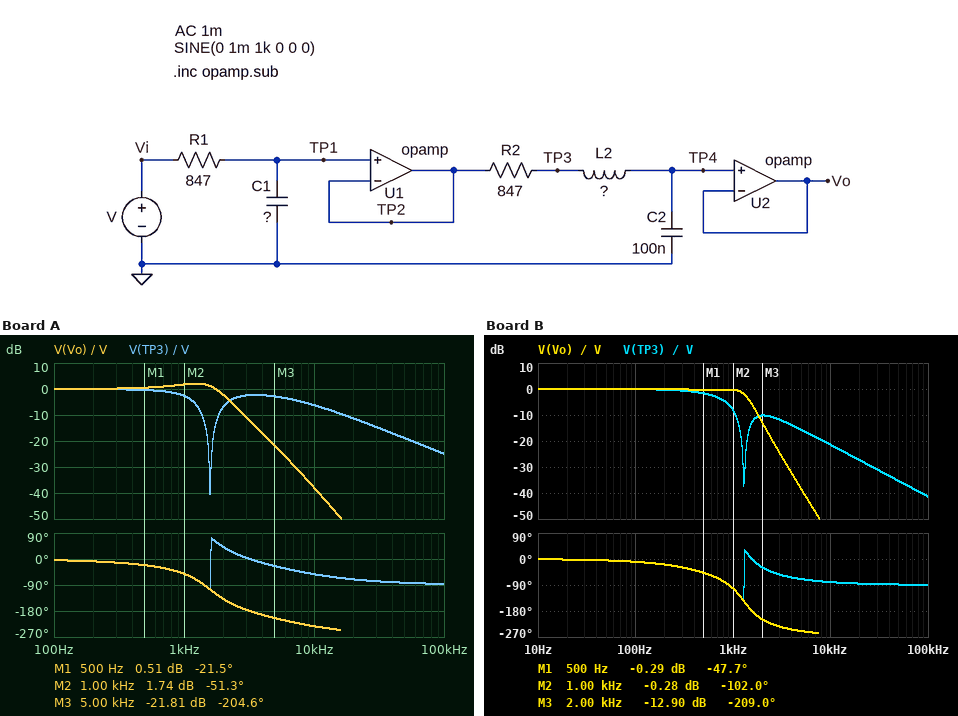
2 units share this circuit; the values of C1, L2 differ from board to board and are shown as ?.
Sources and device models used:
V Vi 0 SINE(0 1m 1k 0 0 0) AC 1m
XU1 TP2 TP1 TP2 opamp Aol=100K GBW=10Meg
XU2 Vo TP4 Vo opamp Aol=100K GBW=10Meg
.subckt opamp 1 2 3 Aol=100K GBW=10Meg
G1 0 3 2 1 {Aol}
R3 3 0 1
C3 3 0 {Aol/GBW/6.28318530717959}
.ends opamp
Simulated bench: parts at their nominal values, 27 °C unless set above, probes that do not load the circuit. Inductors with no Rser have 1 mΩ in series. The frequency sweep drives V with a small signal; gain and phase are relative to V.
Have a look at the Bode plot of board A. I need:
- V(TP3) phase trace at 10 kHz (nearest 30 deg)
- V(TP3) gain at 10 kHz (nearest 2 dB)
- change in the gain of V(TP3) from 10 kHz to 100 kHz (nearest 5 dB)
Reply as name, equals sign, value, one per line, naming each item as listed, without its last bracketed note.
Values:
V(TP3) phase trace at 10 kHz = -60 deg
V(TP3) gain at 10 kHz = -6 dB
change in the gain of V(TP3) from 10 kHz to 100 kHz = -20 dB
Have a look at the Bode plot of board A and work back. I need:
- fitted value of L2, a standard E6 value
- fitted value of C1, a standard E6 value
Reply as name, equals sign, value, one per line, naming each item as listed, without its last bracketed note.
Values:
fitted value of L2, a standard E6 value = 100 mH
fitted value of C1, a standard E6 value = 33 nF
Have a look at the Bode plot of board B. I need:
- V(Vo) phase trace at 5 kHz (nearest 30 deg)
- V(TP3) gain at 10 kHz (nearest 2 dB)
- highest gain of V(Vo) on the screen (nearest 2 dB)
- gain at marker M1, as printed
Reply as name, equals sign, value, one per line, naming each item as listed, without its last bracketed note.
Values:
V(Vo) phase trace at 5 kHz = -240 deg
V(TP3) gain at 10 kHz = -22 dB
highest gain of V(Vo) on the screen = 0 dB
gain at marker M1, as printed = -0.29 dB
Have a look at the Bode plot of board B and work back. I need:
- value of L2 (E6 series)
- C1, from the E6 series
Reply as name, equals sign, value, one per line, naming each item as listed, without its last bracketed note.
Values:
value of L2 = 150 mH
C1, from the E6 series = 220 nF
